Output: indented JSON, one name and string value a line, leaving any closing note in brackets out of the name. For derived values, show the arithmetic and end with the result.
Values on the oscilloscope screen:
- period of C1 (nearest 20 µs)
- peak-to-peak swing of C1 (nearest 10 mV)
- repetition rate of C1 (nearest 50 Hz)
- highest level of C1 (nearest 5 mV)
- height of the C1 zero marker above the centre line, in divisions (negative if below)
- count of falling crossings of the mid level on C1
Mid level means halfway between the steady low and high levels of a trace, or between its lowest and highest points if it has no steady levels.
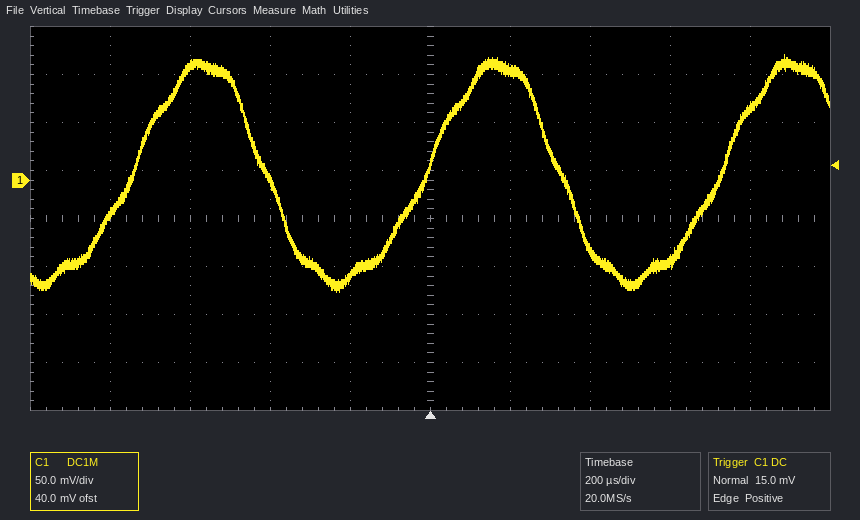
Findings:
{
  "period of C1": "740 µs",
  "peak-to-peak swing of C1": "250 mV",
  "repetition rate of C1": "1 / 740 µs ≈ 1.35 kHz",
  "highest level of C1": "130 mV",
  "height of the C1 zero marker above the centre line, in divisions": "+0.8 div",
  "count of falling crossings of the mid level on C1": "2"
}
